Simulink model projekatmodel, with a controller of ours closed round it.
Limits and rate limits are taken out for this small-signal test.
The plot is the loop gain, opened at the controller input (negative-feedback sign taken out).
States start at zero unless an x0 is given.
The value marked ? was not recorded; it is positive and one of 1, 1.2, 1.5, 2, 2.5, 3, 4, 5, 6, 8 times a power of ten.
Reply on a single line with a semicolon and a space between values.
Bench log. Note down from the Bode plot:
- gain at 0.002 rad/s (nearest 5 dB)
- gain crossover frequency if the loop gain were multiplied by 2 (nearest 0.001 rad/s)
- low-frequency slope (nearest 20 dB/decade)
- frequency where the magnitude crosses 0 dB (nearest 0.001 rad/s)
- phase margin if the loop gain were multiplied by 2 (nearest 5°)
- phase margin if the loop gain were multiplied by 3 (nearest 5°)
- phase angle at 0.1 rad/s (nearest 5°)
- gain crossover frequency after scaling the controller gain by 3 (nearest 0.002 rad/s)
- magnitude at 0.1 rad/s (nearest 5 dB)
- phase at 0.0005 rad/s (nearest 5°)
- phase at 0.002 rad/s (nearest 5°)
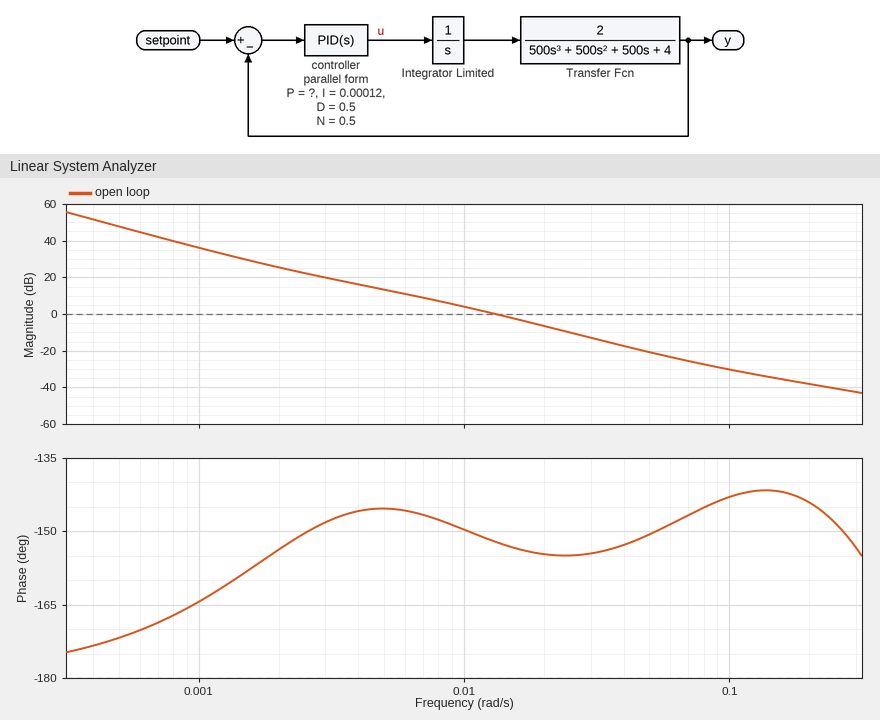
25 dB; 0.019 rad/s; -40 dB/decade; 0.013 rad/s; 25°; 25°; -145°; 0.024 rad/s; -30 dB; -170°; -155°
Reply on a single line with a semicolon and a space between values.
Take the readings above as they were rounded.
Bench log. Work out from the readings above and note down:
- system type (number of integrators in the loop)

2
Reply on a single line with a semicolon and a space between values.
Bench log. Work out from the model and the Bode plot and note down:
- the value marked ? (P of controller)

0.05
